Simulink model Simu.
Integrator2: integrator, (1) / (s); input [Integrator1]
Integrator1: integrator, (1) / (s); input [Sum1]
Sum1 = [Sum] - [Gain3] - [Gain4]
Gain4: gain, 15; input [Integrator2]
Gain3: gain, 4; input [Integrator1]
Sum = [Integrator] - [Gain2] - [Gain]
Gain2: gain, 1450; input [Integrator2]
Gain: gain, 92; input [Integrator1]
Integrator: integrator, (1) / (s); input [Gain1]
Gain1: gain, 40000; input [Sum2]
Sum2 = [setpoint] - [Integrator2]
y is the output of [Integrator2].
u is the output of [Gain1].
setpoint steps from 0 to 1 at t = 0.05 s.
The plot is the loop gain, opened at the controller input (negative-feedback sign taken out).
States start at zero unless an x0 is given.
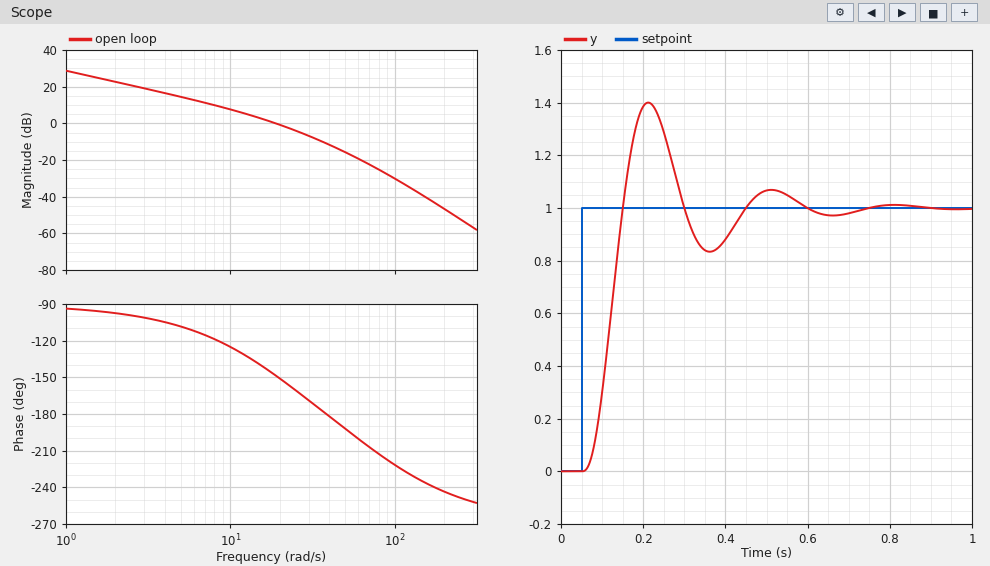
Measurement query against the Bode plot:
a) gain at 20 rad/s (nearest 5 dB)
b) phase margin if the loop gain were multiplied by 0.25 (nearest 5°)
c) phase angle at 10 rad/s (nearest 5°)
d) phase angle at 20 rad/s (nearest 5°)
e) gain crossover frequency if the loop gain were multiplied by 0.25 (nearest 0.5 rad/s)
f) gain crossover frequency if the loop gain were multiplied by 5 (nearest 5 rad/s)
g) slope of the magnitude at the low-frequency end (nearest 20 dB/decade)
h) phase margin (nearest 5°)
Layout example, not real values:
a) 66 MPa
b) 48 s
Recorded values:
a) 0 dB
b) 65°
c) -125°
d) -150°
e) 6.5 rad/s
f) 45 rad/s
g) -20 dB/decade
h) 30°
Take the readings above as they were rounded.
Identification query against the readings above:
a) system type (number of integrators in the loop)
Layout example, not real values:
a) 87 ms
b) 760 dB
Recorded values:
a) 1
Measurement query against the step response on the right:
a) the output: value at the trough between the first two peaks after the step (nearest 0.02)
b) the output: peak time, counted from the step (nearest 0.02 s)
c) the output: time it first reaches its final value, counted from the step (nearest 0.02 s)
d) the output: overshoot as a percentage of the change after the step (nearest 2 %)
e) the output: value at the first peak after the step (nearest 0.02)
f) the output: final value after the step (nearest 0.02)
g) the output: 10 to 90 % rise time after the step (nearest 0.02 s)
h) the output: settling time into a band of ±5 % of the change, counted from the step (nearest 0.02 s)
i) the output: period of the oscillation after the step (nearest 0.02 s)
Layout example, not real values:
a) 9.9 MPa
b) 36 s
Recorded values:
a) 0.84
b) 0.16 s
c) 0.10 s
d) 40 %
e) 1.40
f) 1.00
g) 0.06 s
h) 0.50 s
i) 0.30 s
